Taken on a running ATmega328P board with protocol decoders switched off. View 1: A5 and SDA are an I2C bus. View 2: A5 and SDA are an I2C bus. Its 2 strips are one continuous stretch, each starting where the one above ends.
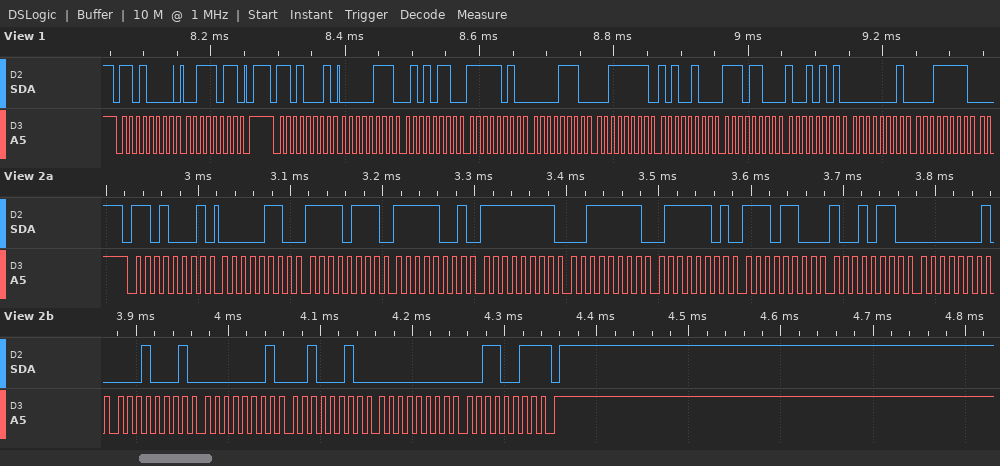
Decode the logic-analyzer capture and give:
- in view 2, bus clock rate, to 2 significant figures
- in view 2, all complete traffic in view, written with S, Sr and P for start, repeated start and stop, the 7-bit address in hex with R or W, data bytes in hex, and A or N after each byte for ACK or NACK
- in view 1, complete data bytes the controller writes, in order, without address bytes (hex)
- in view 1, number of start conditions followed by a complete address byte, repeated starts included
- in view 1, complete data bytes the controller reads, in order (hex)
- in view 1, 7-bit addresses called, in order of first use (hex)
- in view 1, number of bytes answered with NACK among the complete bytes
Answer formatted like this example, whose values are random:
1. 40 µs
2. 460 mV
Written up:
1. 100 kHz
2. S 68R A 06 A F7 A F9 A FF A 3F A 7D A EC A 96 A 01 A 11 A 01 A 22 A 00 A 33 N P
3. 3B
4. 2
5. 07 56 FA 0E 3F A4 EC 95 01 1F
6. 0x68
7. 0
